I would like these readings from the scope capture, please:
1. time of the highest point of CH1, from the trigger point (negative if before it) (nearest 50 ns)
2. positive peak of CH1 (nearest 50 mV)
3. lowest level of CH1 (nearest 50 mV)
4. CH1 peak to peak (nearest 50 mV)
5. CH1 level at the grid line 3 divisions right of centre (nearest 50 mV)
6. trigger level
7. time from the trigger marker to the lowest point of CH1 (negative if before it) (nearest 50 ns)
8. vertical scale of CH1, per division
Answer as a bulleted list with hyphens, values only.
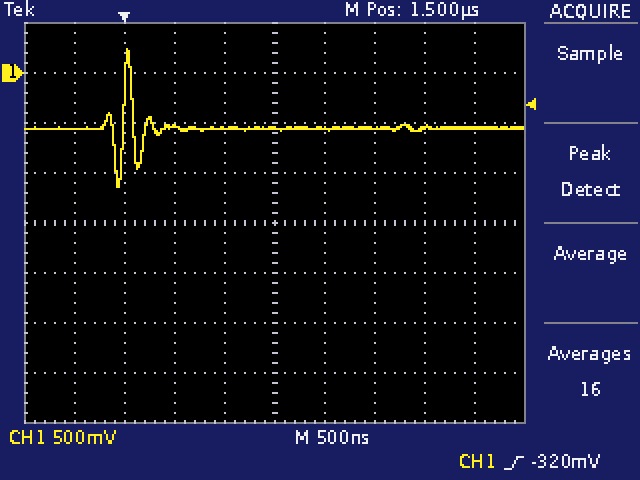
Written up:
- +50 ns
- 250 mV
- -1.15 V
- 1.40 V
- -550 mV
- -320 mV
- -50 ns
- 500 mV
